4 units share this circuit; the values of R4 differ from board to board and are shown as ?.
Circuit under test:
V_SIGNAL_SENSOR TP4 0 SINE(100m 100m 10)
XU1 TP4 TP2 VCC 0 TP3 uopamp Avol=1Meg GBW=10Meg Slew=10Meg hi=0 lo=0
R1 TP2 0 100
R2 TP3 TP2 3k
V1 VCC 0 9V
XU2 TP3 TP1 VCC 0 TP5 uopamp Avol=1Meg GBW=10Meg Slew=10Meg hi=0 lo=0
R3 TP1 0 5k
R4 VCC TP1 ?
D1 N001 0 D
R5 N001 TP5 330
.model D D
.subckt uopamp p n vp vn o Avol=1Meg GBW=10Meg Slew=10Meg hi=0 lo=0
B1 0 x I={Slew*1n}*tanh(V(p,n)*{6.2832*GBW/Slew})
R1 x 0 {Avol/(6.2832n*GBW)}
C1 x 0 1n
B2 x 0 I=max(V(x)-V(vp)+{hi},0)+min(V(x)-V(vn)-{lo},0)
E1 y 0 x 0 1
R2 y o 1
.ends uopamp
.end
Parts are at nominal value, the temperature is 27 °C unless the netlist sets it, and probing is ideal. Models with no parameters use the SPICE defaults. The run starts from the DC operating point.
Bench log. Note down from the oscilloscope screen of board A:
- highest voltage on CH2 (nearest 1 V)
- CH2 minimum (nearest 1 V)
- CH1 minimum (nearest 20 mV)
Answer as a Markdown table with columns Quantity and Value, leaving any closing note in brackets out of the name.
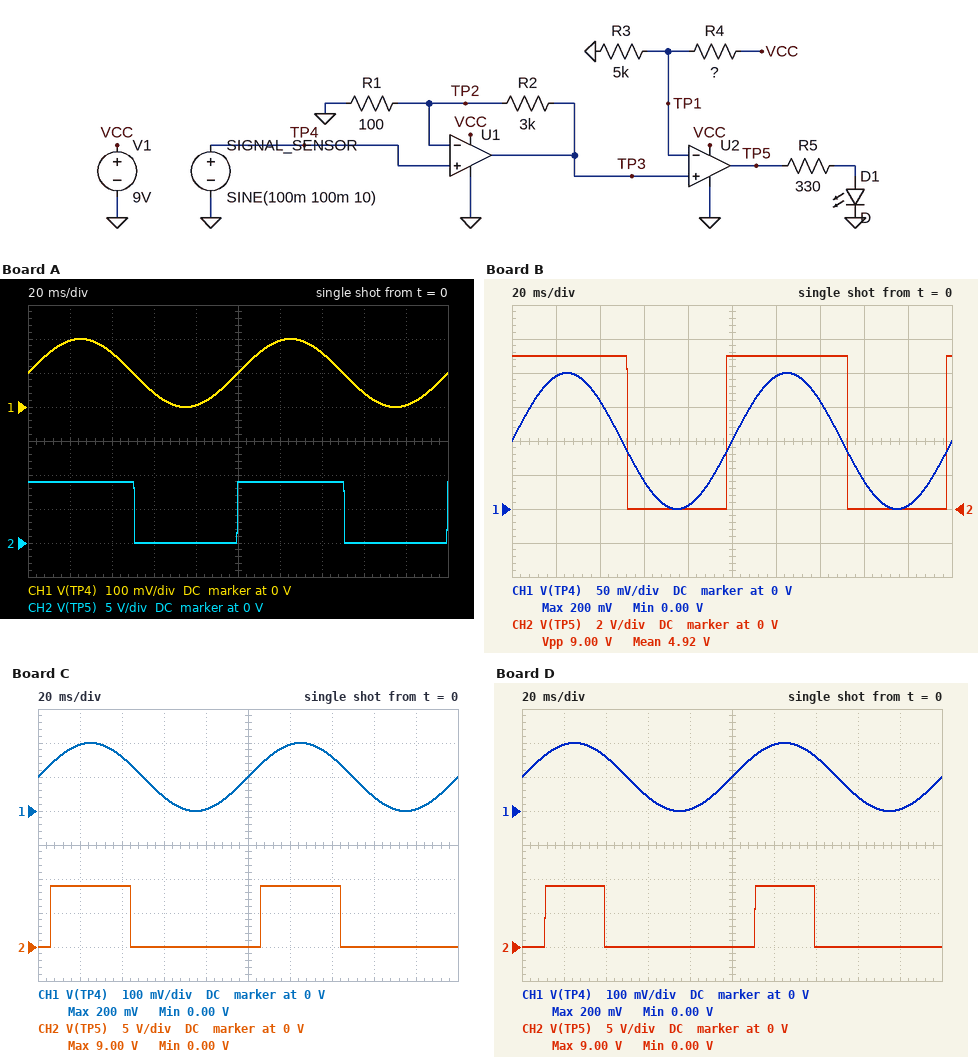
| Quantity | Value |
|---|---|
| highest voltage on CH2 | 9 V |
| CH2 minimum | 0 V |
| CH1 minimum | 0 V |
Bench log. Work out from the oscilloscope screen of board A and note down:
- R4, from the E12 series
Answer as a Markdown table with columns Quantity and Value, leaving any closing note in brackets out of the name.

| Quantity | Value |
|---|---|
| R4, from the E12 series | 10 kΩ |
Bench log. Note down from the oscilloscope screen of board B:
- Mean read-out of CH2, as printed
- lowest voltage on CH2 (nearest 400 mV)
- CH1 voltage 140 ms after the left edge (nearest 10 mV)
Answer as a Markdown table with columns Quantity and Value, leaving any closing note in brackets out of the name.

| Quantity | Value |
|---|---|
| Mean read-out of CH2, as printed | 4.92 V |
| lowest voltage on CH2 | 0 V |
| CH1 voltage 140 ms after the left edge | 160 mV |
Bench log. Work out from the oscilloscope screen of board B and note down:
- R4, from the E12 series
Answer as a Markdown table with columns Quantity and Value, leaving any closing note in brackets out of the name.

| Quantity | Value |
|---|---|
| R4, from the E12 series | 12 kΩ |
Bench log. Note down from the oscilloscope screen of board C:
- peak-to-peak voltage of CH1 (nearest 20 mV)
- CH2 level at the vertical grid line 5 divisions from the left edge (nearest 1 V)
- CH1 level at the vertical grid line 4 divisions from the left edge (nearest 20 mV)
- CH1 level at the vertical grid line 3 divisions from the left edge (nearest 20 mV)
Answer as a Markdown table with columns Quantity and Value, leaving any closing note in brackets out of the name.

| Quantity | Value |
|---|---|
| peak-to-peak voltage of CH1 | 200 mV |
| CH2 level at the vertical grid line 5 divisions from the left edge | 0 V |
| CH1 level at the vertical grid line 4 divisions from the left edge | 0 V |
| CH1 level at the vertical grid line 3 divisions from the left edge | 40 mV |
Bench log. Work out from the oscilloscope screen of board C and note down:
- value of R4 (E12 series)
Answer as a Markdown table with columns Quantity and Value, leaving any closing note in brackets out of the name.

| Quantity | Value |
|---|---|
| value of R4 | 5.6 kΩ |
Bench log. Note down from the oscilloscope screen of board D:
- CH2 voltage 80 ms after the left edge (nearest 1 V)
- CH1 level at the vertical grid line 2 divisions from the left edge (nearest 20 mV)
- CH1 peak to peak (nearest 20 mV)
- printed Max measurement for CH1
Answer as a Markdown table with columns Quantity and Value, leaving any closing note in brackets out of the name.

| Quantity | Value |
|---|---|
| CH2 voltage 80 ms after the left edge | 0 V |
| CH1 level at the vertical grid line 2 divisions from the left edge | 160 mV |
| CH1 peak to peak | 200 mV |
| printed Max measurement for CH1 | 200 mV |
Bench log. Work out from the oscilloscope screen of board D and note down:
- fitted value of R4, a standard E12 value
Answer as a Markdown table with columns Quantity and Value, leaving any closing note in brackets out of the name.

| Quantity | Value |
|---|---|
| fitted value of R4, a standard E12 value | 3.9 kΩ |
